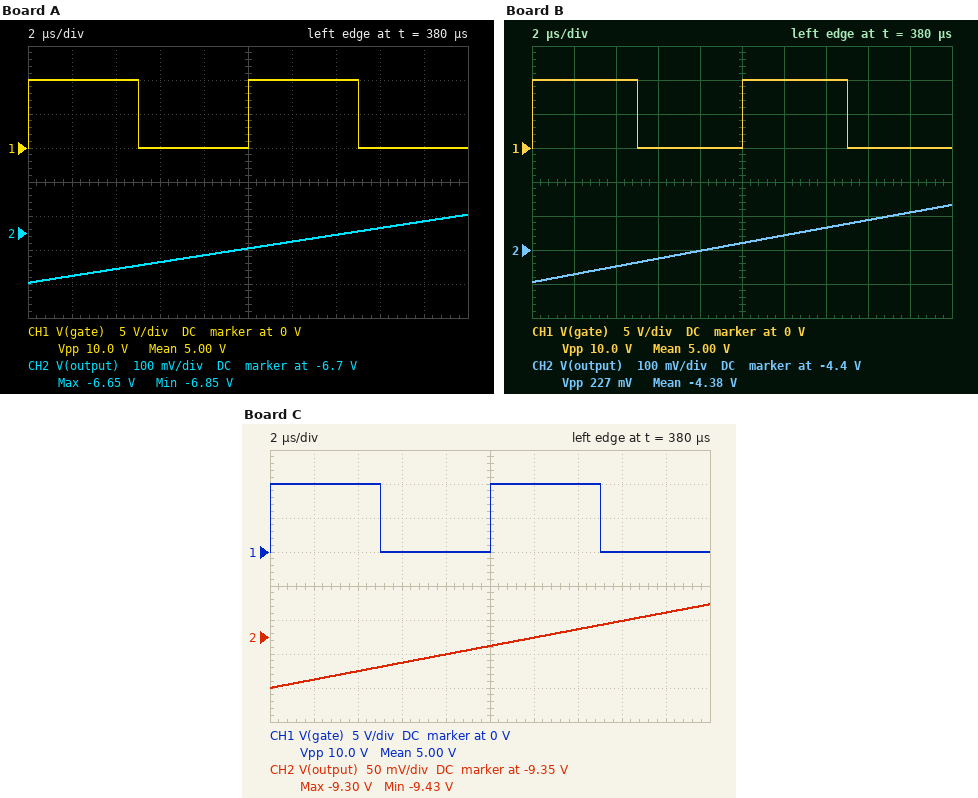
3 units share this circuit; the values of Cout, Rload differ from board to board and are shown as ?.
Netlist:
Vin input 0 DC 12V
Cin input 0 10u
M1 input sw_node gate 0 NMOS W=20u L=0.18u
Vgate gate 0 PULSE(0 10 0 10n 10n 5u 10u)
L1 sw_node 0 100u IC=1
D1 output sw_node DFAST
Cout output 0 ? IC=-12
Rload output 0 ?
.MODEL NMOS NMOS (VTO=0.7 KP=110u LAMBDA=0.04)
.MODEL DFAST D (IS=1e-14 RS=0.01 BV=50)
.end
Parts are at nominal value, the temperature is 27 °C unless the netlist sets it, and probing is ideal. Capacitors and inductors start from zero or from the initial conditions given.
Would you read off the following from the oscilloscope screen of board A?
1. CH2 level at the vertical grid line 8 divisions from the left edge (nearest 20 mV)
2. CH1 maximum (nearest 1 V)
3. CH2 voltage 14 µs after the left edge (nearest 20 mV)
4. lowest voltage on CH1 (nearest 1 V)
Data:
-6.68 V
10 V
-6.70 V
0 V
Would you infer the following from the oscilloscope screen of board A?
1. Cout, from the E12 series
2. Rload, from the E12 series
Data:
82 µF
8.2 Ω
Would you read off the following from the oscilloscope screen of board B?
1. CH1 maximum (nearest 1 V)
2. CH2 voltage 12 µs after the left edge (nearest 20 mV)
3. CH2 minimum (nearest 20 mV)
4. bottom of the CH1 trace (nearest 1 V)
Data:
10 V
-4.36 V
-4.50 V
0 V
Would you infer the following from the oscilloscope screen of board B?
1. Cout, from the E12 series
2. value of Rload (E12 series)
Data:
82 µF
4.7 Ω
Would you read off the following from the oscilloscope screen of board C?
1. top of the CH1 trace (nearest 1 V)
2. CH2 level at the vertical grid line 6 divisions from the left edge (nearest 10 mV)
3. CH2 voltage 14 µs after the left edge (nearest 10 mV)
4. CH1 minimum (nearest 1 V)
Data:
10 V
-9.35 V
-9.34 V
0 V
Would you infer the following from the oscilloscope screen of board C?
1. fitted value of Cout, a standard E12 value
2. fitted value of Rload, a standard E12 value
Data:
39 µF
39 Ω
